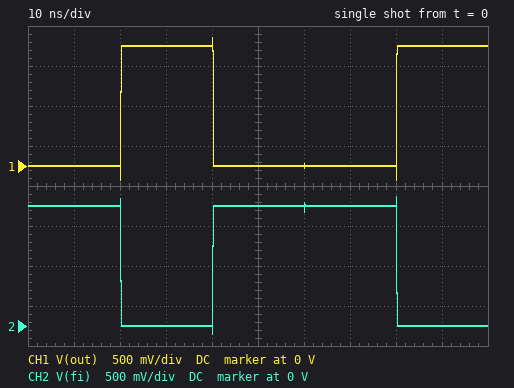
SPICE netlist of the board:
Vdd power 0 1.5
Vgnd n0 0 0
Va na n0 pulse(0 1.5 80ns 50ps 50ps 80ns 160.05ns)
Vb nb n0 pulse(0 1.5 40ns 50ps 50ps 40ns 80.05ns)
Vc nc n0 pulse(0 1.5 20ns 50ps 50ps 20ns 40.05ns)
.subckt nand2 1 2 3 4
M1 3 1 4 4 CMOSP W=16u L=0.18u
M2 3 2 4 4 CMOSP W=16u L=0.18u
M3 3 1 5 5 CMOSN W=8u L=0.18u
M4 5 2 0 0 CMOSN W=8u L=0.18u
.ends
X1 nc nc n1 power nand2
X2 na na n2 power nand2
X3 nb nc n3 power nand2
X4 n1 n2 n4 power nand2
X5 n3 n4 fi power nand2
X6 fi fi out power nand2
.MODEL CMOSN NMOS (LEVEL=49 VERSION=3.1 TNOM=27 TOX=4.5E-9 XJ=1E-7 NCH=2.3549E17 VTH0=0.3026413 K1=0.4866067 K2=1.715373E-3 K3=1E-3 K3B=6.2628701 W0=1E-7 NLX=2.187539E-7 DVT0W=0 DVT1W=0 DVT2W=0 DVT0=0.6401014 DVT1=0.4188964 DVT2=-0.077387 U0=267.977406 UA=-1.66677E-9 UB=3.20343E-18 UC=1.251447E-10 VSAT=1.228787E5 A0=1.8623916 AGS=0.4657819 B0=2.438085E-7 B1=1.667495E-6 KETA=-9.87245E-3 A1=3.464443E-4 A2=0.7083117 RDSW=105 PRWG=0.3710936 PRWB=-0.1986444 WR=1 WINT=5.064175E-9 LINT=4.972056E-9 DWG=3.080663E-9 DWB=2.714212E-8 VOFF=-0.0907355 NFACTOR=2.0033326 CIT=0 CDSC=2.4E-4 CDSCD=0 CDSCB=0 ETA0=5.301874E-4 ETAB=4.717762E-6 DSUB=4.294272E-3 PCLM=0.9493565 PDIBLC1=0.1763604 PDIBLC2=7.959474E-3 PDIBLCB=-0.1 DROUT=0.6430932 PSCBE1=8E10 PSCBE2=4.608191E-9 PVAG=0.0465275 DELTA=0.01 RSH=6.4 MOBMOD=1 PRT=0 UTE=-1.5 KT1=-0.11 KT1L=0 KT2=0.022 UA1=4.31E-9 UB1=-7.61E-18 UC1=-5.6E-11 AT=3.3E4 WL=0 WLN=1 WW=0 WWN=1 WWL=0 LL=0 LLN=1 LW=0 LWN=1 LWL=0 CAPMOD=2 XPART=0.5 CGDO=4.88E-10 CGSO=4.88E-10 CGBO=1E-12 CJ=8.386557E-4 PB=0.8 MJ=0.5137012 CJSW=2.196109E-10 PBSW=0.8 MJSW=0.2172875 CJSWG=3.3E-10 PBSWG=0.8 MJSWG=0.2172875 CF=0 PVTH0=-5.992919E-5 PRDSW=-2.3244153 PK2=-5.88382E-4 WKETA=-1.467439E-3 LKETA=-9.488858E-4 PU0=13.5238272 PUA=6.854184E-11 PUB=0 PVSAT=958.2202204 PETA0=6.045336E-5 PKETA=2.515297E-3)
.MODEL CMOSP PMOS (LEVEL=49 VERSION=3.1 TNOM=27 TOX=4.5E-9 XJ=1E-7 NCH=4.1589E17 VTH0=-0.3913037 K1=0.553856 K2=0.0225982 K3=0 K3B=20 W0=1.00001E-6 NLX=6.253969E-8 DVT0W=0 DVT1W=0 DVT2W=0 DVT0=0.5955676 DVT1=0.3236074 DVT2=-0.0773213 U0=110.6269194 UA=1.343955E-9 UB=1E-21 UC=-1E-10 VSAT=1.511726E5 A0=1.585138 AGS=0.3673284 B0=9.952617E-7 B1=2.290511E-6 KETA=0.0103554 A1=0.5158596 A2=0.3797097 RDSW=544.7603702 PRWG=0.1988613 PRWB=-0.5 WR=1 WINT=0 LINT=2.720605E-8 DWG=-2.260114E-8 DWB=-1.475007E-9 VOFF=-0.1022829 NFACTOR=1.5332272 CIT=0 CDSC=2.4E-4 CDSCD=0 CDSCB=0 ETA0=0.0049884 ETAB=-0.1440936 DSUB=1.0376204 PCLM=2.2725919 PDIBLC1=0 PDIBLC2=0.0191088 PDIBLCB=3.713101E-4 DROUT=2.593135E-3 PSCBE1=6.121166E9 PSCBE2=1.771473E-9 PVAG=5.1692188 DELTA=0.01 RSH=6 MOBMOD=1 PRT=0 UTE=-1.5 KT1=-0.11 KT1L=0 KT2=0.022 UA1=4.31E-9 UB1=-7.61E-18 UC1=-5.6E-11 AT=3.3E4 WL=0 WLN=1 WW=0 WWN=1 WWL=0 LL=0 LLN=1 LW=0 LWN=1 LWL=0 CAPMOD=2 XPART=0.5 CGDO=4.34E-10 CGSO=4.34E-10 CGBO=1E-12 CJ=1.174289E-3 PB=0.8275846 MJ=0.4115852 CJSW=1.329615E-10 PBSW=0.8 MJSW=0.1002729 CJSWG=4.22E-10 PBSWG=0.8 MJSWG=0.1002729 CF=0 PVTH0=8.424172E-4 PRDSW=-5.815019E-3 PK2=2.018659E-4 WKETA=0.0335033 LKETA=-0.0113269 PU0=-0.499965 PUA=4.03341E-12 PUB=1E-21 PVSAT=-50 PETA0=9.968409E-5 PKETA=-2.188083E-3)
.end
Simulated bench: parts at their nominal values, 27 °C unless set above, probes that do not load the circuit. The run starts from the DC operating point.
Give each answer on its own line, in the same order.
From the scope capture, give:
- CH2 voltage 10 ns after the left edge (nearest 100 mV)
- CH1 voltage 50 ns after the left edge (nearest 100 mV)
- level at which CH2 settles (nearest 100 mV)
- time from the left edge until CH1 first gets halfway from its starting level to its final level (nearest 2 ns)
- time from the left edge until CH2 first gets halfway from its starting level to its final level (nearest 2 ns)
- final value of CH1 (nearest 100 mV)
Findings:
1.5 V
0 V
0 V
20 ns
20 ns
1.5 V
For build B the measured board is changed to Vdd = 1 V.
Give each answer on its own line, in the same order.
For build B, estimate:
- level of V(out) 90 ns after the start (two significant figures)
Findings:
1.0 V
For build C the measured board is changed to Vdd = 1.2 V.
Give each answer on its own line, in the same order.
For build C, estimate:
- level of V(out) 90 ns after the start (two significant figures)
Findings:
1.2 V
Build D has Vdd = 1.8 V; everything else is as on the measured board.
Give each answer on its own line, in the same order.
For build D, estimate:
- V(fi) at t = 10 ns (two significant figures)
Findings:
1.8 V
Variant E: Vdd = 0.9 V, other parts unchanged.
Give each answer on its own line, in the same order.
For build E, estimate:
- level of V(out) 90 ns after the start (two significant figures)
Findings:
900 mV
